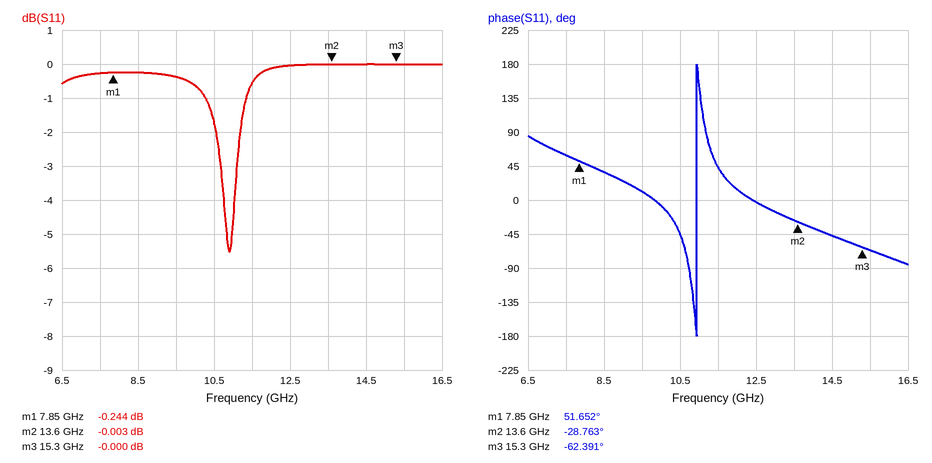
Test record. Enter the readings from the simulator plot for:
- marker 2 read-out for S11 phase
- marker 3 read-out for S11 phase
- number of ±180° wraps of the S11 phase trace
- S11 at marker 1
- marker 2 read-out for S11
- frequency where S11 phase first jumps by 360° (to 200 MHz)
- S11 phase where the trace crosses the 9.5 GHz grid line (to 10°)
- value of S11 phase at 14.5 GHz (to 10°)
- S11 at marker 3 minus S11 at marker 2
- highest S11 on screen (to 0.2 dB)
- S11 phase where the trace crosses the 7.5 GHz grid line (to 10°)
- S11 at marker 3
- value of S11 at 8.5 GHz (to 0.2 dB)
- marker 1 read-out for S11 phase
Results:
-28.763°
-62.391°
1
-0.244 dB
-0.003 dB
11.0 GHz
10°
-50°
0.003 dB
0.0 dB
60°
-0.000 dB
-0.2 dB
51.652°
